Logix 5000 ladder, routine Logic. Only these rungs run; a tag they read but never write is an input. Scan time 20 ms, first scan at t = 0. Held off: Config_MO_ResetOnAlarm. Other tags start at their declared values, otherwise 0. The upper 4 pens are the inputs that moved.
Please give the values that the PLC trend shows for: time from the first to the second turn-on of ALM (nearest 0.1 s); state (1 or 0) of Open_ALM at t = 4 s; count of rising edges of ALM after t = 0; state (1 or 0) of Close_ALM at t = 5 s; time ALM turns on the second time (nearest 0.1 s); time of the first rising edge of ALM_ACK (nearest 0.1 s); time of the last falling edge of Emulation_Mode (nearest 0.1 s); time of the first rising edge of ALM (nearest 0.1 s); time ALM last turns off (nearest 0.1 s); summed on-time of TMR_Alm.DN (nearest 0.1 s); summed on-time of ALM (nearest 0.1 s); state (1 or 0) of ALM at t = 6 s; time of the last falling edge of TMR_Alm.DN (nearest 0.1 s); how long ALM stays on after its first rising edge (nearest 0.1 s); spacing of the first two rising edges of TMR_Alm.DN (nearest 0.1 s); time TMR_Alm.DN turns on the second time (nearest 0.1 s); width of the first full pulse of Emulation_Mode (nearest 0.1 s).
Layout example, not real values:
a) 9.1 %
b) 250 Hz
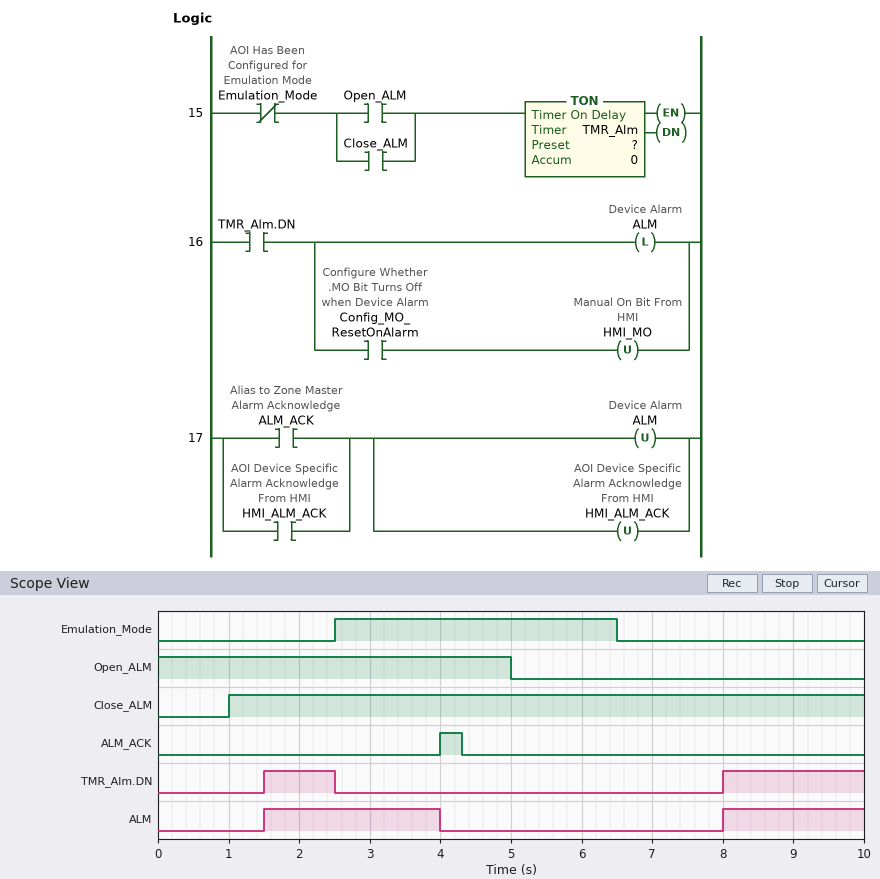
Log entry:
a) 6.5 s
b) 1
c) 2
d) 1
e) 8.0 s
f) 4.0 s
g) 6.5 s
h) 1.5 s
i) 4.0 s
j) 3.0 s
k) 4.5 s
l) 0
m) 2.5 s
n) 2.5 s
o) 6.5 s
p) 8.0 s
q) 4.0 s
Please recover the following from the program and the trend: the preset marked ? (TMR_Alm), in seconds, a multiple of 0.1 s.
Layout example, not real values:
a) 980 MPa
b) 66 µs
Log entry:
a) 1.5 s
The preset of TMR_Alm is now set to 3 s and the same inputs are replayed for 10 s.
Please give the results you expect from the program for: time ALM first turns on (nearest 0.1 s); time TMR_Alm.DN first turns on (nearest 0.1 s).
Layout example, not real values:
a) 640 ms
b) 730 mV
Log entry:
a) 9.5 s
b) 9.5 s
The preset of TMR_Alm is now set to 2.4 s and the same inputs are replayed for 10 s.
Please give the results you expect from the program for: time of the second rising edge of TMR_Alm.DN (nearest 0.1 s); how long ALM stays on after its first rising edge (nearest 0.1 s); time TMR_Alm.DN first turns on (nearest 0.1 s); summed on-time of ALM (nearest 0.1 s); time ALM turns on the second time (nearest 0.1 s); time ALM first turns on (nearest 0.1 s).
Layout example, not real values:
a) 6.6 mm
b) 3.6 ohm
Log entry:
a) 8.9 s
b) 1.6 s
c) 2.4 s
d) 2.7 s
e) 8.9 s
f) 2.4 s
